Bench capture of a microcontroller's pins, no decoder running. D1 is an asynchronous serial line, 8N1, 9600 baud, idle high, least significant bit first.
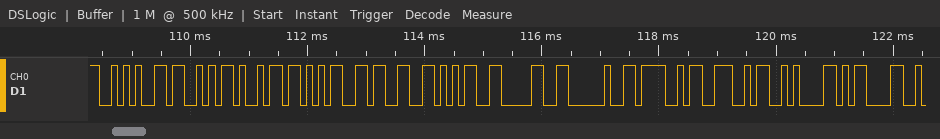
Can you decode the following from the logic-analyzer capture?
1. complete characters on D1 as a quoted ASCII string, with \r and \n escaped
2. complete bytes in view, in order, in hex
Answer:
"*Si5350 ON\n\r"
0x2A 0x53 0x69 0x35 0x33 0x35 0x30 0x20 0x4F 0x4E 0x0A 0x0D
